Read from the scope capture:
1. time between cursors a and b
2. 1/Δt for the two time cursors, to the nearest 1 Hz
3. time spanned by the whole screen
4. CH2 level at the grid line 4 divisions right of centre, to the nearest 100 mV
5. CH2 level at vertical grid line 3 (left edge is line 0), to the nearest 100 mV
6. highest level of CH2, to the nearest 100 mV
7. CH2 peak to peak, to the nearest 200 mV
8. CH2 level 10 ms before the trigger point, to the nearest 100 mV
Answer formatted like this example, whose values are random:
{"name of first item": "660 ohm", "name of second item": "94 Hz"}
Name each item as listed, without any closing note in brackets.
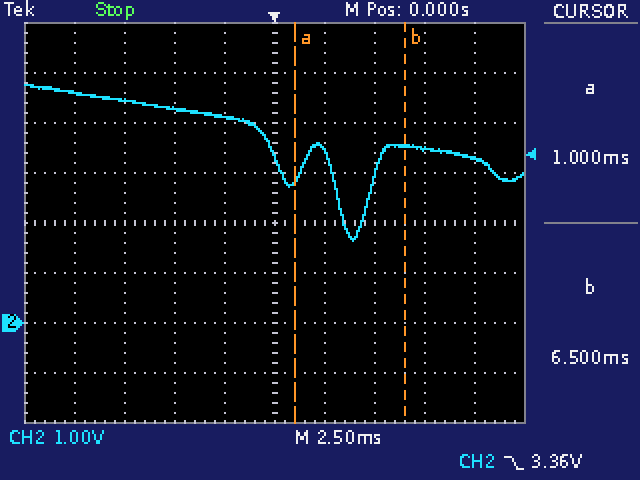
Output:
{"time between cursors a and b": "5.50 ms", "1/Δt for the two time cursors, to the nearest 1 Hz": "182 Hz", "time spanned by the whole screen": "25 ms", "CH2 level at the grid line 4 divisions right of centre, to the nearest 100 mV": "3.3 V", "CH2 level at vertical grid line 3 (left edge is line 0), to the nearest 100 mV": "4.3 V", "highest level of CH2, to the nearest 100 mV": "4.8 V", "CH2 peak to peak, to the nearest 200 mV": "3.2 V", "CH2 level 10 ms before the trigger point, to the nearest 100 mV": "4.6 V"}
